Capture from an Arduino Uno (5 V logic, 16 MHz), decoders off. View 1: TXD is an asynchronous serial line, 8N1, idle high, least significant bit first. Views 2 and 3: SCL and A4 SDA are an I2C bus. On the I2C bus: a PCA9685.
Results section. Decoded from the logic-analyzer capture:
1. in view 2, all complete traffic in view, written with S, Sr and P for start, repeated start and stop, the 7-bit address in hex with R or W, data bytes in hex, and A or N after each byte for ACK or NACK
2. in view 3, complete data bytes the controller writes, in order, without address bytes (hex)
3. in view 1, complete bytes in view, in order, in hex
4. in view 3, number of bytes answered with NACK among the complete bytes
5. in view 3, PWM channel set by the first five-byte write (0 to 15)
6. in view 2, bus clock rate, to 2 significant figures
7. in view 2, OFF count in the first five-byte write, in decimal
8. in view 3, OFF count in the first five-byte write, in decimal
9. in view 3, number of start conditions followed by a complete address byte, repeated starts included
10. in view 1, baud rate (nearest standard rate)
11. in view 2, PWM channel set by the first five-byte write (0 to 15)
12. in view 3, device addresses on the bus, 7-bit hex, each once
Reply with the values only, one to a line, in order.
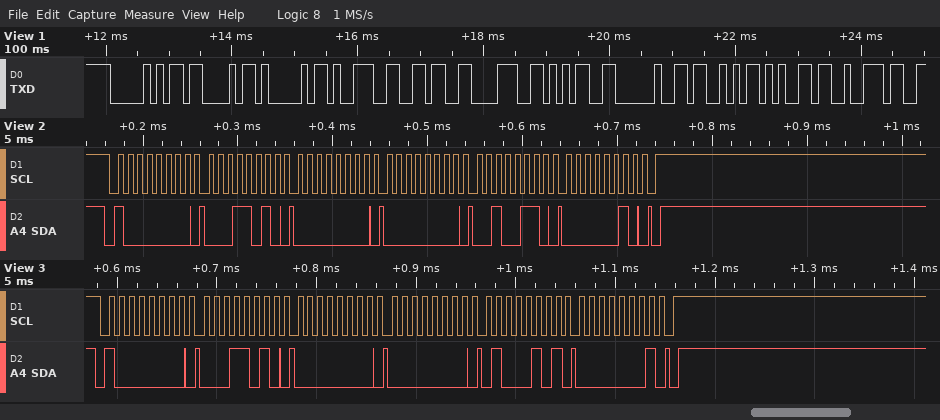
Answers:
S 40W A 1A A 00 A 00 A 26 A 02 A P
1A 00 00 45 01
50 43 41 39 36 38 35 20 53 65 72
0
5
100 kHz
550
325
1
9600 baud
5
0x40
